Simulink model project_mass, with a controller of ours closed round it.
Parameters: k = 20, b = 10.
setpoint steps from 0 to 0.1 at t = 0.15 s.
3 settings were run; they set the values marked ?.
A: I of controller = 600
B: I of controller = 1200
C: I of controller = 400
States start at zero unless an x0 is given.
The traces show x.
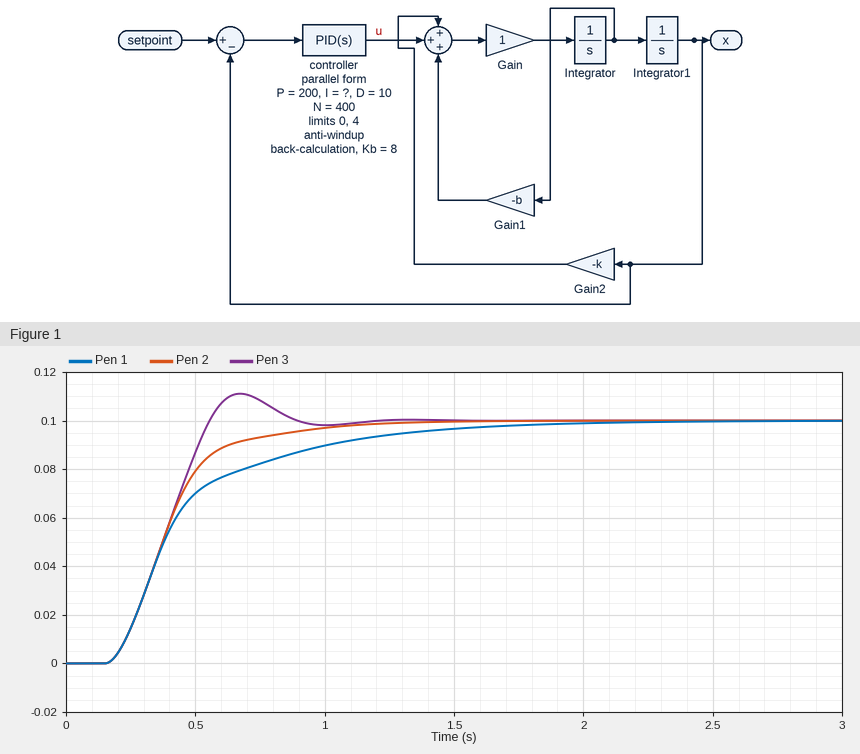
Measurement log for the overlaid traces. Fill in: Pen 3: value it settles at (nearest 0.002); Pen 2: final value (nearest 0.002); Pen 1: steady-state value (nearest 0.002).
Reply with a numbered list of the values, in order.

1. 0.100
2. 0.100
3. 0.100
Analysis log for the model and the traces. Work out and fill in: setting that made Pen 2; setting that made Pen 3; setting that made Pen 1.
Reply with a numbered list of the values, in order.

1. A
2. B
3. C
